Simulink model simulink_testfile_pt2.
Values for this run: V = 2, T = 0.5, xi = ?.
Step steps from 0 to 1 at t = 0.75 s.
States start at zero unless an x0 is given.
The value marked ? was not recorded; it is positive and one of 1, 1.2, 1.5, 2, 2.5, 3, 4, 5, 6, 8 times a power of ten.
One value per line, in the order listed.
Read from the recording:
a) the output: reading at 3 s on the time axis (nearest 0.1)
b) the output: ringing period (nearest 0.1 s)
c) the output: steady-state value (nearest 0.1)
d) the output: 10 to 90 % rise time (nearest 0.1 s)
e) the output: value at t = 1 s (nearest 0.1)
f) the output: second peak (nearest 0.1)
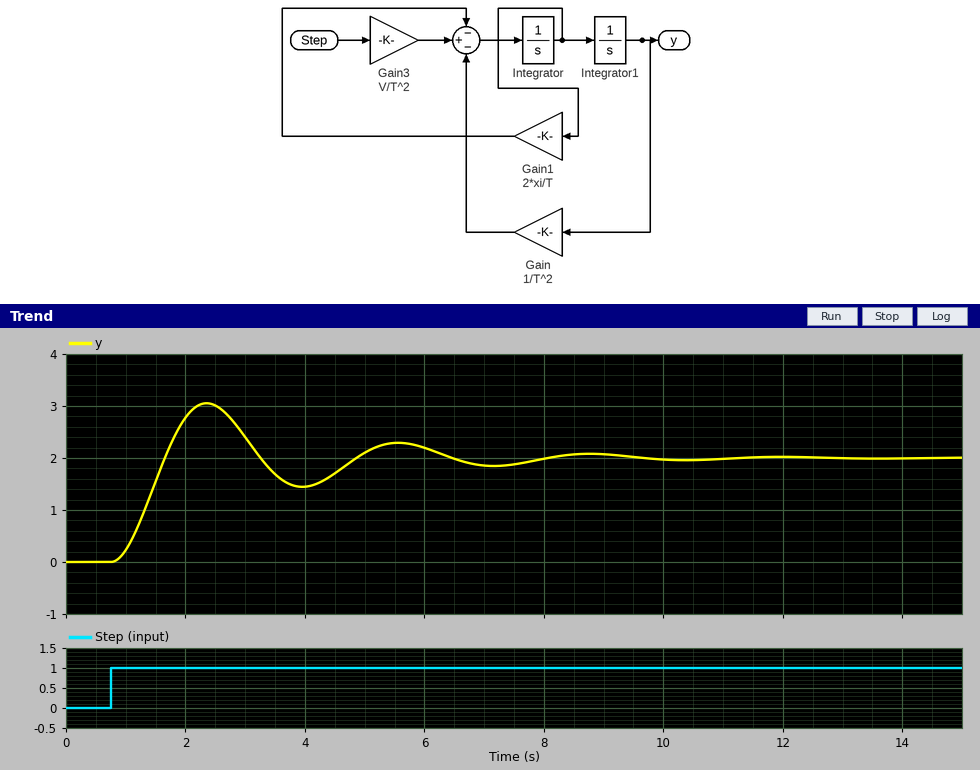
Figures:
2.4
3.2 s
2.0
0.6 s
0.2
2.3
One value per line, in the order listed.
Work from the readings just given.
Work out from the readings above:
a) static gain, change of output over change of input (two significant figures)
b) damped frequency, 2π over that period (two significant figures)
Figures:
2.0
2.0 rad/s
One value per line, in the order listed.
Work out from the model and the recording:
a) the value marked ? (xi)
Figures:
0.2
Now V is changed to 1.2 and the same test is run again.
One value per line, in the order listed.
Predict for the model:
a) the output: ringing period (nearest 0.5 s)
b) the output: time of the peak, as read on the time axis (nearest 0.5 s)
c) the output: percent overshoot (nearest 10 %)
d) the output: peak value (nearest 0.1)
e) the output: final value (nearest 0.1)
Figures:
3.0 s
2.5 s
50 %
1.8
1.2
